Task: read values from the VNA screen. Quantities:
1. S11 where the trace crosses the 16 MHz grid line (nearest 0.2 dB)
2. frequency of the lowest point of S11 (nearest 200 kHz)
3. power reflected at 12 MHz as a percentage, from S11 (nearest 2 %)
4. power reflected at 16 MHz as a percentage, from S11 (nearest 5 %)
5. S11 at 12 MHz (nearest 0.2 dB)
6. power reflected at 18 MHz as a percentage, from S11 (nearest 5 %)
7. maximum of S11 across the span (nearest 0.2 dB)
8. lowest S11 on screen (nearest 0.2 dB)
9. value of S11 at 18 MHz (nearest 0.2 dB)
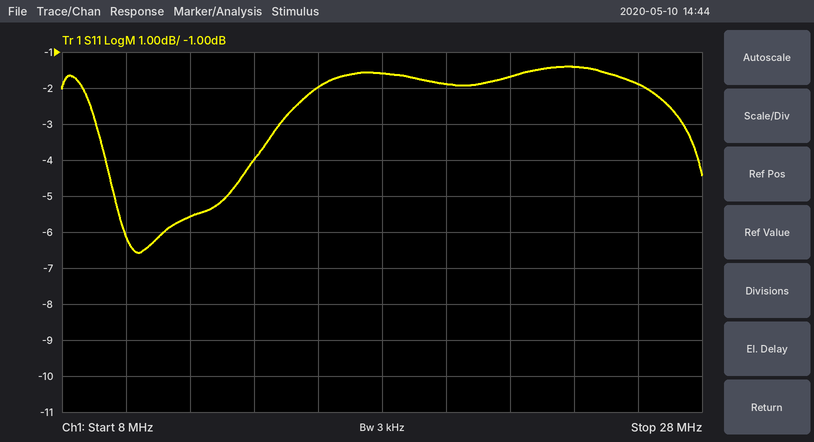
-2.0 dB
10.4 MHz
28 %
65 %
-5.6 dB
70 %
-1.4 dB
-6.6 dB
-1.6 dB
